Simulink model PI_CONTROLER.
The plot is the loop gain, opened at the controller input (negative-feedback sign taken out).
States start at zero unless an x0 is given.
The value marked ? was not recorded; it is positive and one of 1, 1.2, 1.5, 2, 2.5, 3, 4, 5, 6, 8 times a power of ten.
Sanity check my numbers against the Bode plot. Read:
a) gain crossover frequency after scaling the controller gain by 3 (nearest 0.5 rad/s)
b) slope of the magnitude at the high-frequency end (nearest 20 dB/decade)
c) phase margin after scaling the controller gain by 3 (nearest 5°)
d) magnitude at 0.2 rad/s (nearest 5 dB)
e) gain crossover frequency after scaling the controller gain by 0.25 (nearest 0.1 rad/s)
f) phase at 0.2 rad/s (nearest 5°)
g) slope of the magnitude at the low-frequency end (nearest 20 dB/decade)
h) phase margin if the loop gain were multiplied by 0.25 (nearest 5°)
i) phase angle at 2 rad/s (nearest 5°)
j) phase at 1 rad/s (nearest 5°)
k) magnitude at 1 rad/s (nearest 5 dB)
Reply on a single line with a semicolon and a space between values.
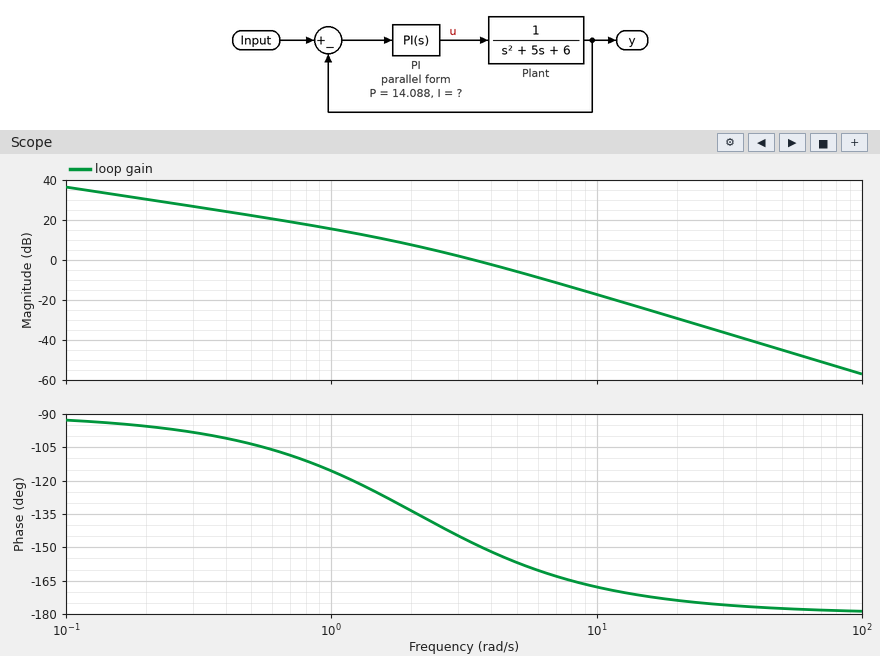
6.5 rad/s; -40 dB/decade; 20°; 30 dB; 1.4 rad/s; -95°; -20 dB/decade; 55°; -135°; -115°; 15 dB
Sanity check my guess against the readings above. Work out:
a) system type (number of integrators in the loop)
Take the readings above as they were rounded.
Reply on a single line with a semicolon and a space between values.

1
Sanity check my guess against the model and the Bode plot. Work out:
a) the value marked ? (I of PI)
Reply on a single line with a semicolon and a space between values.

40
